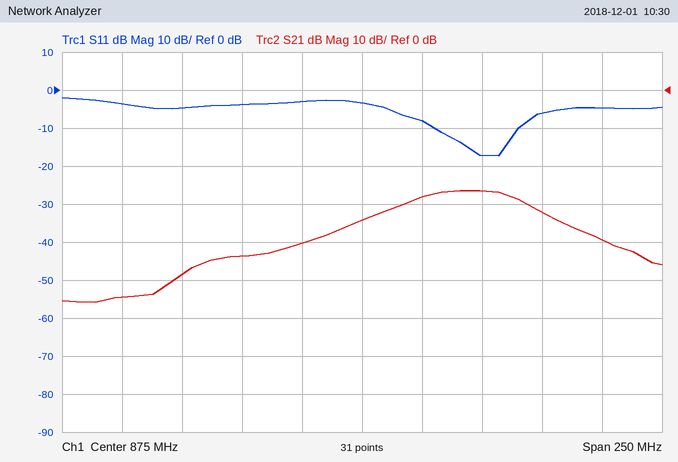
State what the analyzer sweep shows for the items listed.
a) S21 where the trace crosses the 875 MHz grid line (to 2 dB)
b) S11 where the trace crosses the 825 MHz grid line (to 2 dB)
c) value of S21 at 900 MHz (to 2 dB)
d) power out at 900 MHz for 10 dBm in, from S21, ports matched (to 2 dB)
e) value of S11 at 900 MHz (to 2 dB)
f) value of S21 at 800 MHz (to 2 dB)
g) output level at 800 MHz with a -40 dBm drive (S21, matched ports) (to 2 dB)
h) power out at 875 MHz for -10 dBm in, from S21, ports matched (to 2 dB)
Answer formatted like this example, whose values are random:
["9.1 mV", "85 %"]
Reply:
["-34 dB", "-4 dB", "-28 dB", "-18 dBm", "-8 dB", "-48 dB", "-88 dBm", "-44 dBm"]
